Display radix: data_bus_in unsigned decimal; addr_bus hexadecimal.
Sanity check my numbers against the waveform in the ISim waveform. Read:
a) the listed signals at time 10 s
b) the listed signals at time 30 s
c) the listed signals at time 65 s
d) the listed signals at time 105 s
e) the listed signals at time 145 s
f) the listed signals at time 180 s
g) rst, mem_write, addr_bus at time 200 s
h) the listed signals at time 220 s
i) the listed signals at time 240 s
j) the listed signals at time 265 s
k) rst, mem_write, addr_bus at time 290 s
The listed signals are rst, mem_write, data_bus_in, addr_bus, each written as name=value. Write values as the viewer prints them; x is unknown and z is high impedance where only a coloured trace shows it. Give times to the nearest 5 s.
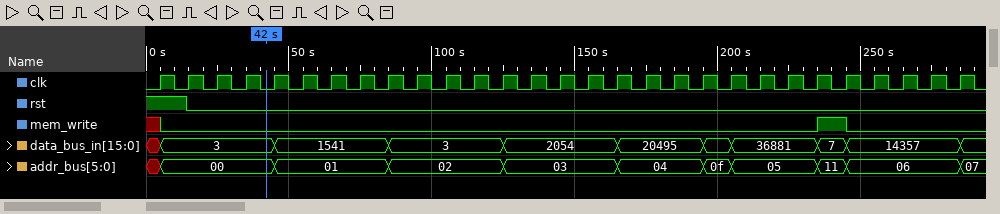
rst=1, mem_write=0, data_bus_in=3, addr_bus=00
rst=0, mem_write=0, data_bus_in=3, addr_bus=00
rst=0, mem_write=0, data_bus_in=1541, addr_bus=01
rst=0, mem_write=0, data_bus_in=3, addr_bus=02
rst=0, mem_write=0, data_bus_in=2054, addr_bus=03
rst=0, mem_write=0, data_bus_in=20495, addr_bus=04
rst=0, mem_write=0, addr_bus=0f
rst=0, mem_write=0, data_bus_in=36881, addr_bus=05
rst=0, mem_write=1, data_bus_in=7, addr_bus=11
rst=0, mem_write=0, data_bus_in=14357, addr_bus=06
rst=0, mem_write=0, addr_bus=07
